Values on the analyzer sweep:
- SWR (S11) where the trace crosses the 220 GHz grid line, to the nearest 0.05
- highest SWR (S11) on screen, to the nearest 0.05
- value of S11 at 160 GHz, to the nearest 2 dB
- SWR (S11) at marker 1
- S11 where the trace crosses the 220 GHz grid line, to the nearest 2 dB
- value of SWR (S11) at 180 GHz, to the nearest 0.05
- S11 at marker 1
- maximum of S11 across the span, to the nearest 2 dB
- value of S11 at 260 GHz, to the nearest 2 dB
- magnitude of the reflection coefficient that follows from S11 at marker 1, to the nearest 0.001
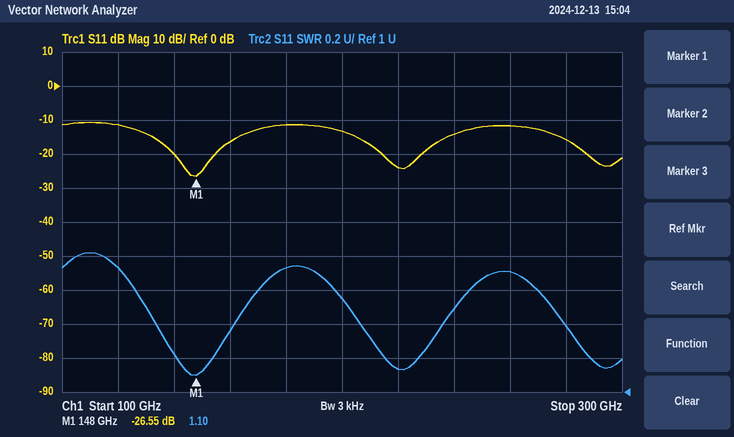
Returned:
1.15
1.80
-16 dB
1.10
-24 dB
1.75
-26.55 dB
-10 dB
-12 dB
0.047
